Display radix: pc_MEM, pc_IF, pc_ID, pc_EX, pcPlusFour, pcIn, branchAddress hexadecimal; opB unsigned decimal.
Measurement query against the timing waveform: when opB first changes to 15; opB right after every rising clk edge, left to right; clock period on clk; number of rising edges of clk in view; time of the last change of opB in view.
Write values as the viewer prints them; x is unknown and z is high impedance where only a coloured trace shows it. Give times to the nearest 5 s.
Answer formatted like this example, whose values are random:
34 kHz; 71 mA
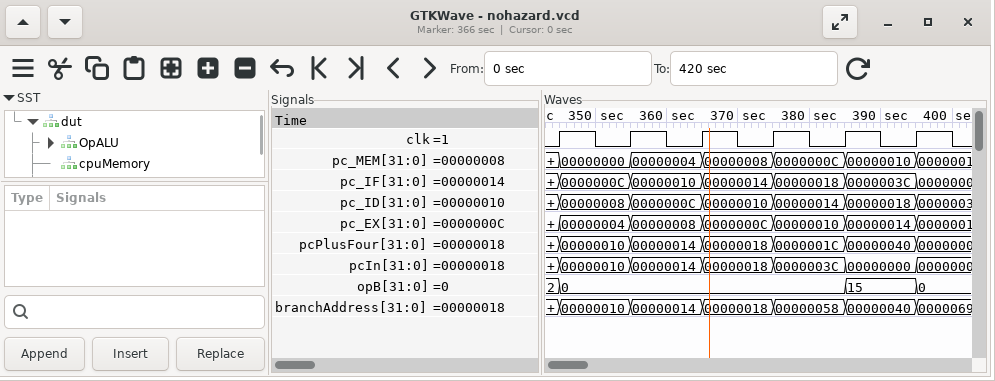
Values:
385 s; 0, 0, 0, 0, 15, 0; 10 s; 6; 395 s
